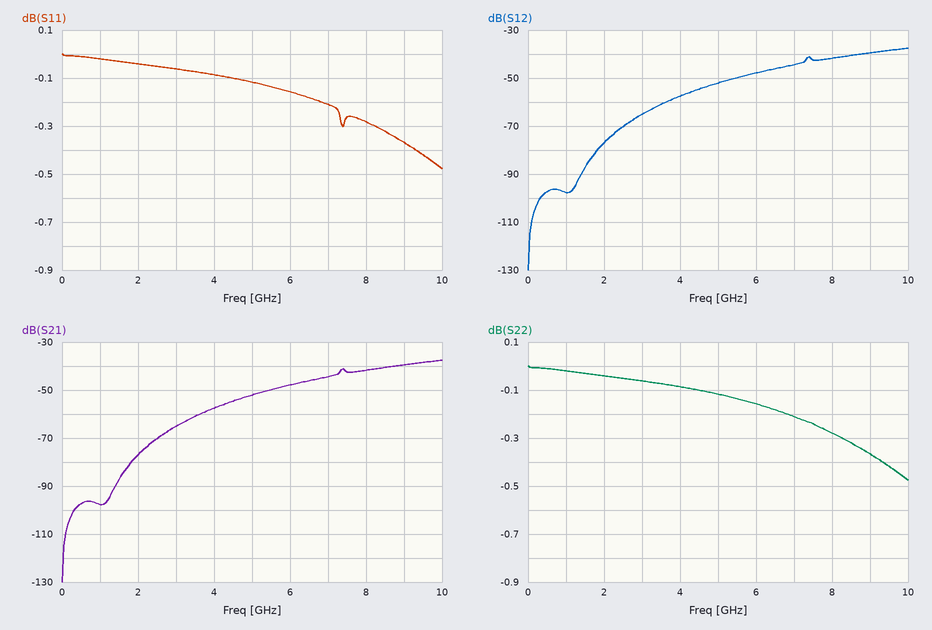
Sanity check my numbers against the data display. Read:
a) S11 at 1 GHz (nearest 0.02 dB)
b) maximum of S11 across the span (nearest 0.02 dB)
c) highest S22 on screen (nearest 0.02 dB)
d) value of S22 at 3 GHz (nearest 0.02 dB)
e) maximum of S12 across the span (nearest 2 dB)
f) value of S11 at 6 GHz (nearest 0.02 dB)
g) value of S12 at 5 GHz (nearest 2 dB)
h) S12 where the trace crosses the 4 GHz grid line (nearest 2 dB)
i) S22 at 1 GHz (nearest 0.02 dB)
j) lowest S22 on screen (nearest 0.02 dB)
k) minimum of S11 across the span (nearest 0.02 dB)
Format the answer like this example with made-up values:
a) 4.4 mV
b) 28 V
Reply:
a) -0.02 dB
b) 0.00 dB
c) 0.00 dB
d) -0.06 dB
e) -38 dB
f) -0.16 dB
g) -52 dB
h) -58 dB
i) -0.02 dB
j) -0.48 dB
k) -0.48 dB
